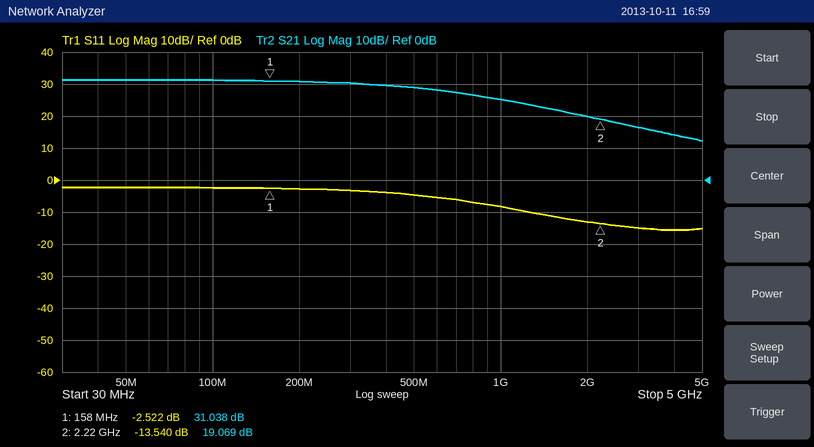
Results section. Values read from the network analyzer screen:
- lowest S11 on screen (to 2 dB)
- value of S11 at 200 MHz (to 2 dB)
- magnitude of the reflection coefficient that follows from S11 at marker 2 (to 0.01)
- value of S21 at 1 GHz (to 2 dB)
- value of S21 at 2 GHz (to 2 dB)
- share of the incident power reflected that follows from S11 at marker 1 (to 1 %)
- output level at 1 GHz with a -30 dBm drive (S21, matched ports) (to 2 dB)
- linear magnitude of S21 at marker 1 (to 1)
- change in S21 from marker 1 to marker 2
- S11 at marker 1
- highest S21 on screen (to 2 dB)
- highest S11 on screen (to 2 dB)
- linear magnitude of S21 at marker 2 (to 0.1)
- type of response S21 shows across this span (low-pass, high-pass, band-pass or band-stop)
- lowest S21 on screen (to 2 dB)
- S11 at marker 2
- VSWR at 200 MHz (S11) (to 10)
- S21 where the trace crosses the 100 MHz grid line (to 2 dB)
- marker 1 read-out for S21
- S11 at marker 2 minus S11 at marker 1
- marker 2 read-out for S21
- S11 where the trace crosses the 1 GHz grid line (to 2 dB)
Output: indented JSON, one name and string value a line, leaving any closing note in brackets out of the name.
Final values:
{
  "lowest S11 on screen": "-16 dB",
  "value of S11 at 200 MHz": "-2 dB",
  "magnitude of the reflection coefficient that follows from S11 at marker 2": "0.21",
  "value of S21 at 1 GHz": "26 dB",
  "value of S21 at 2 GHz": "20 dB",
  "share of the incident power reflected that follows from S11 at marker 1": "56 %",
  "output level at 1 GHz with a -30 dBm drive (S21, matched ports)": "-4 dBm",
  "linear magnitude of S21 at marker 1": "36",
  "change in S21 from marker 1 to marker 2": "-11.969 dB",
  "S11 at marker 1": "-2.522 dB",
  "highest S21 on screen": "32 dB",
  "highest S11 on screen": "-2 dB",
  "linear magnitude of S21 at marker 2": "9.0",
  "type of response S21 shows across this span": "low-pass",
  "lowest S21 on screen": "12 dB",
  "S11 at marker 2": "-13.540 dB",
  "VSWR at 200 MHz (S11)": "10",
  "S21 where the trace crosses the 100 MHz grid line": "32 dB",
  "marker 1 read-out for S21": "31.038 dB",
  "S11 at marker 2 minus S11 at marker 1": "-11.018 dB",
  "marker 2 read-out for S21": "19.069 dB",
  "S11 where the trace crosses the 1 GHz grid line": "-8 dB"
}
